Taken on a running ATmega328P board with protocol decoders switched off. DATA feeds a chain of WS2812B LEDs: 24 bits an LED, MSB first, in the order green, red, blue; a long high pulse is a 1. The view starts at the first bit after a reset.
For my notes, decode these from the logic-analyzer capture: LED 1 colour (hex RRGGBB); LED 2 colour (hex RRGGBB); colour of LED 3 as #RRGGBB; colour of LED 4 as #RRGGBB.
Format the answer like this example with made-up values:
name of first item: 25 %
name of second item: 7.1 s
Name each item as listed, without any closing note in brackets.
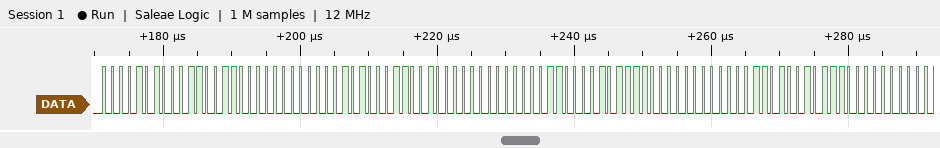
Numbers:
LED 1 colour: #330A00
LED 2 colour: #320A00
colour of LED 3 as #RRGGBB: #2F0C00
colour of LED 4 as #RRGGBB: #2E0D00
